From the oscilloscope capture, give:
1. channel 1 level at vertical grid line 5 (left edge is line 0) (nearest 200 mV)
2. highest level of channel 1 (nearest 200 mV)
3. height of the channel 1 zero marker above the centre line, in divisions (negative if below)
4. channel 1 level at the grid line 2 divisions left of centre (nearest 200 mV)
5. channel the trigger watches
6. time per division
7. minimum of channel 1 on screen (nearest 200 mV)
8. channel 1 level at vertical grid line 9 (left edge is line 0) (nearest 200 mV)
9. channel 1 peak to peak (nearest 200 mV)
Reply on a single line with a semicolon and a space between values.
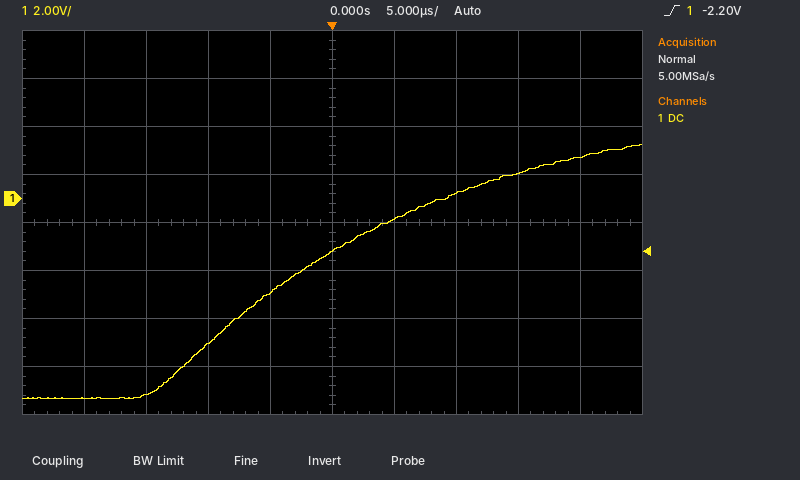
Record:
-2.2 V; 2.2 V; +0.5 div; -6.0 V; channel 1; 5 µs; -8.4 V; 1.8 V; 10.6 V
